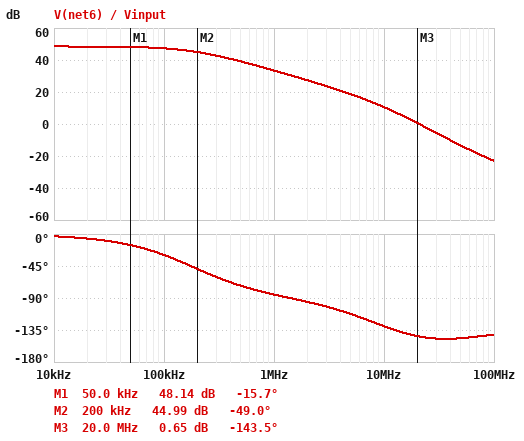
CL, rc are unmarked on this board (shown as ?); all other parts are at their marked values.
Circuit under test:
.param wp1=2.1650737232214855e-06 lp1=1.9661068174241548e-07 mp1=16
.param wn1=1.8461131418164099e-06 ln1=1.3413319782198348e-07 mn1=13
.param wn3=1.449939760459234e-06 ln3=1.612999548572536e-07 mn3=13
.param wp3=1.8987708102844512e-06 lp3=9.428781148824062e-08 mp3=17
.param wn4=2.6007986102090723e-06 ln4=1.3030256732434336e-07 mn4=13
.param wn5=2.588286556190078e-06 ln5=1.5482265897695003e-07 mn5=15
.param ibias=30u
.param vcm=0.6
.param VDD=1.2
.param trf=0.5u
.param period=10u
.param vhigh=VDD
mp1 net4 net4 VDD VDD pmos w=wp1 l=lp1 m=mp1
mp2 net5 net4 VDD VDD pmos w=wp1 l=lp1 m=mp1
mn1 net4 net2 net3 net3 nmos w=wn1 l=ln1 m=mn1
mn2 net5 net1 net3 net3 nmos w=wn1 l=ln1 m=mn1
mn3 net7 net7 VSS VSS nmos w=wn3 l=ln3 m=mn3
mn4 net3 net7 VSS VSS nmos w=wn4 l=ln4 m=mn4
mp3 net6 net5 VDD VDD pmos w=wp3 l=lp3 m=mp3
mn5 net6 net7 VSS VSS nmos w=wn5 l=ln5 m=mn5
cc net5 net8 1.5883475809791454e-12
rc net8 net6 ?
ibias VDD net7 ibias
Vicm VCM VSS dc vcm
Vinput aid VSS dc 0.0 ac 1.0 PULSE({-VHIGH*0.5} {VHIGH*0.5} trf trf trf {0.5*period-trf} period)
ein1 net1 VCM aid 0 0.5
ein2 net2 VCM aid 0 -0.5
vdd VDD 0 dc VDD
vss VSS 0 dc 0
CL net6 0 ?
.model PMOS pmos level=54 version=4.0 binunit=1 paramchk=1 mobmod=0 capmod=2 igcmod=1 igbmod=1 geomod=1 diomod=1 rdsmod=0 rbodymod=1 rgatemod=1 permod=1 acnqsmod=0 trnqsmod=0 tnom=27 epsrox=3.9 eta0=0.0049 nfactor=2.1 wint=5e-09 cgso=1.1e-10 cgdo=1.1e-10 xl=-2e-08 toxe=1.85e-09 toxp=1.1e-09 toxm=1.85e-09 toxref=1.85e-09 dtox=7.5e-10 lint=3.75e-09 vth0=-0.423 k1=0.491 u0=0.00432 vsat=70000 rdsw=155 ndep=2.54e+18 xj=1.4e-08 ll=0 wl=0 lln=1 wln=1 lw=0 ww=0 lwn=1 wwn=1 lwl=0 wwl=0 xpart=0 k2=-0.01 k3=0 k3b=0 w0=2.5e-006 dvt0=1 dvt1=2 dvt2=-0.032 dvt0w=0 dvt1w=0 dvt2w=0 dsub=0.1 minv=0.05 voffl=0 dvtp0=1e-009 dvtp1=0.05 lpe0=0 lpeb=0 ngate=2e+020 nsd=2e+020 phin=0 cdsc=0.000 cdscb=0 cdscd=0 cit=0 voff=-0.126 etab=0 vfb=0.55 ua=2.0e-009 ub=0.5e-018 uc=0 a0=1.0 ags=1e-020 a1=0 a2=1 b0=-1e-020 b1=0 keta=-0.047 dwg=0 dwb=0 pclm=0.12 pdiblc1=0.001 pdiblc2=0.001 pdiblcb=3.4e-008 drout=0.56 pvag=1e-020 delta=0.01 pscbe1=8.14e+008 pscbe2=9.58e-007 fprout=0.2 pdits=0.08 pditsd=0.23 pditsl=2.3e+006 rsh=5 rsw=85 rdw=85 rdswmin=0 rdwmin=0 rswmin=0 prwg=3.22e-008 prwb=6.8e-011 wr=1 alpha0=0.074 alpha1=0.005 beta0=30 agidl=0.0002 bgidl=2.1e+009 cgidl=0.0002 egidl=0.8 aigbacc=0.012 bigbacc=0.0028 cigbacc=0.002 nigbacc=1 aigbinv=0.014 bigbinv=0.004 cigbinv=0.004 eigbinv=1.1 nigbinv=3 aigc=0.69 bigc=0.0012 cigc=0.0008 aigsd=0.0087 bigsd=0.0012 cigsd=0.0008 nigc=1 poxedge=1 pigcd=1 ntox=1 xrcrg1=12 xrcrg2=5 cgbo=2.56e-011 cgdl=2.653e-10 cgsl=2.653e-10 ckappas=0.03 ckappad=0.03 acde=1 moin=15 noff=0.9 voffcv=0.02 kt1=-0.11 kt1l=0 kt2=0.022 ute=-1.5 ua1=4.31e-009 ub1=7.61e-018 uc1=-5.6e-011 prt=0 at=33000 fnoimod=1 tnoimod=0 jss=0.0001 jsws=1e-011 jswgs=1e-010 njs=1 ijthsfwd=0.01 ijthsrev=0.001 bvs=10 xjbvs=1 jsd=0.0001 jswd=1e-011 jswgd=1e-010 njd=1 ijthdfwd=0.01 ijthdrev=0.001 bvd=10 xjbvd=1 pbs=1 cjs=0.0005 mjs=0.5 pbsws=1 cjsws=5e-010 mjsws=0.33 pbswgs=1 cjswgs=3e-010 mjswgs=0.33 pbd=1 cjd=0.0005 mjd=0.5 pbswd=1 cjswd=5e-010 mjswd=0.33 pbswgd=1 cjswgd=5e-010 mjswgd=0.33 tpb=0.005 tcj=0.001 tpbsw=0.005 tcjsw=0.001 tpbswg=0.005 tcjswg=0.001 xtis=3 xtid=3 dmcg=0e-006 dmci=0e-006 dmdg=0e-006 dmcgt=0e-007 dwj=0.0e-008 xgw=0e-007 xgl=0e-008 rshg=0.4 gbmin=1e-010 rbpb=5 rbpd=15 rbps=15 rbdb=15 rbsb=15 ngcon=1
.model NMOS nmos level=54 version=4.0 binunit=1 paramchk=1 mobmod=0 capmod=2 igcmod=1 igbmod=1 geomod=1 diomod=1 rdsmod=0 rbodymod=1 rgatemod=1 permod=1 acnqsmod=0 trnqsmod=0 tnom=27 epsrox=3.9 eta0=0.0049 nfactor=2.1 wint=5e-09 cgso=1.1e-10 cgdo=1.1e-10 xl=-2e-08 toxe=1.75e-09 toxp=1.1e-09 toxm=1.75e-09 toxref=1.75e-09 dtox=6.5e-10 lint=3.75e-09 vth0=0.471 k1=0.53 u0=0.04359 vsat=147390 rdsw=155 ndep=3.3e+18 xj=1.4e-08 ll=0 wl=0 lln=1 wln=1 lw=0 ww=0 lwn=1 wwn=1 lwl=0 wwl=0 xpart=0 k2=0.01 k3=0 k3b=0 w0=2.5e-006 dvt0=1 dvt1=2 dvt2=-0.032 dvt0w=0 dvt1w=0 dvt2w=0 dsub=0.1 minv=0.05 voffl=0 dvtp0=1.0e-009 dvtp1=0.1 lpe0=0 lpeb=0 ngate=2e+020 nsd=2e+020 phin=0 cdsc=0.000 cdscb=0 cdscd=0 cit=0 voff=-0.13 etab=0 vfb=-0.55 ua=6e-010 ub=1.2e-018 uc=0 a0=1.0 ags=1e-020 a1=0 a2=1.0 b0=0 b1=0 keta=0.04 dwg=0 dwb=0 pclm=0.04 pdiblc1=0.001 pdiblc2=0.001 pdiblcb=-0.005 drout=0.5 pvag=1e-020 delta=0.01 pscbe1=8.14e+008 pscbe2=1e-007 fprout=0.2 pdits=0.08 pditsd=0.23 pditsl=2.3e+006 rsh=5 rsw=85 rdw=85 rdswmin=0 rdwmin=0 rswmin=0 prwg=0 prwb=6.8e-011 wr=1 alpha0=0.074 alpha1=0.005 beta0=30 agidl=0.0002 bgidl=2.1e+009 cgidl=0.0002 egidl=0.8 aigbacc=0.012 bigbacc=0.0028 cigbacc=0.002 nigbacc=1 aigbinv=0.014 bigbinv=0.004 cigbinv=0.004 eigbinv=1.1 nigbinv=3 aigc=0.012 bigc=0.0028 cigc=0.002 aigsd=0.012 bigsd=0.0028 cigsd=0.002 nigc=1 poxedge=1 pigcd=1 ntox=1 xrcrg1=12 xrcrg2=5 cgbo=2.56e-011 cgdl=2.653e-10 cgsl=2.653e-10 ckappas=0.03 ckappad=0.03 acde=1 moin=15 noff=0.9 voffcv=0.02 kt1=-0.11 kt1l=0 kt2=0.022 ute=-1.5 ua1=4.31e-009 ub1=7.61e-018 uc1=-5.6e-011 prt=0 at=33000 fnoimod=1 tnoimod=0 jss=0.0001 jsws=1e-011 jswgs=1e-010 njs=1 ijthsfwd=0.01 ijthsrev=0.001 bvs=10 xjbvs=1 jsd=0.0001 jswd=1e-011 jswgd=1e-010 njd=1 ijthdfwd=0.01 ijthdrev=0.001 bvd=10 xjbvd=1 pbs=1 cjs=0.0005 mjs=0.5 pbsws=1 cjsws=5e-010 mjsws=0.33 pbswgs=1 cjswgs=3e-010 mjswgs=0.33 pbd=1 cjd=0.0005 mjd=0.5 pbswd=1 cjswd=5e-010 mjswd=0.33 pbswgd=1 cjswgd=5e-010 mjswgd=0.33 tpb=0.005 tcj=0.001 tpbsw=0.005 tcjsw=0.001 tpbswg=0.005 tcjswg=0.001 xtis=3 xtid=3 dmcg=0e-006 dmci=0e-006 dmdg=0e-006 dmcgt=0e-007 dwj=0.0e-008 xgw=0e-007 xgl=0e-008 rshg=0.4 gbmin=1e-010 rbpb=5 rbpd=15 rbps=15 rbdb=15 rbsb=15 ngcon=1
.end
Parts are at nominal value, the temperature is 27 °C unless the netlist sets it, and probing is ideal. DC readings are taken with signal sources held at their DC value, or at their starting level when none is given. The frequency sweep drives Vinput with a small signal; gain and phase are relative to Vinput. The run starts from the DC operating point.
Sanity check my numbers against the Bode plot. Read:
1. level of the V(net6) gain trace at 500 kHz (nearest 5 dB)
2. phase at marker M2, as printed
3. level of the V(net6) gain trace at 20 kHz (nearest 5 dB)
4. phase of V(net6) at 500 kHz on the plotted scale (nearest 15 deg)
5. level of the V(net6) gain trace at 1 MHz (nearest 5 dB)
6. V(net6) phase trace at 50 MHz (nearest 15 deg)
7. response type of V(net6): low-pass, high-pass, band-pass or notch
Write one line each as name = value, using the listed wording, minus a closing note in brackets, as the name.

level of the V(net6) gain trace at 500 kHz = 40 dB
phase at marker M2, as printed = -49.0 deg
level of the V(net6) gain trace at 20 kHz = 50 dB
phase of V(net6) at 500 kHz on the plotted scale = -75 deg
level of the V(net6) gain trace at 1 MHz = 35 dB
V(net6) phase trace at 50 MHz = -150 deg
response type of V(net6): low-pass, high-pass, band-pass or notch = low-pass
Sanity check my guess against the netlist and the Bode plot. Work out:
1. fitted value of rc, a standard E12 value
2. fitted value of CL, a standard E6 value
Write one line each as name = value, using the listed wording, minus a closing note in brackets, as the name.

fitted value of rc, a standard E12 value = 2.2 kΩ
fitted value of CL, a standard E6 value = 22 pF
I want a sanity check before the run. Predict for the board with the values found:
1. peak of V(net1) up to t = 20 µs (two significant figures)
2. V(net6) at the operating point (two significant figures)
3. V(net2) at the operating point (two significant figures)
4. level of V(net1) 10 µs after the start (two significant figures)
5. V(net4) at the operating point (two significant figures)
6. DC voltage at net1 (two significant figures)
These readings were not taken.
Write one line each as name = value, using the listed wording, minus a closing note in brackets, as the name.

peak of V(net1) up to t = 20 µs = 900 mV
V(net6) at the operating point = 1.1 V
V(net2) at the operating point = 600 mV
level of V(net1) 10 µs after the start = 300 mV
V(net4) at the operating point = 720 mV
DC voltage at net1 = 600 mV
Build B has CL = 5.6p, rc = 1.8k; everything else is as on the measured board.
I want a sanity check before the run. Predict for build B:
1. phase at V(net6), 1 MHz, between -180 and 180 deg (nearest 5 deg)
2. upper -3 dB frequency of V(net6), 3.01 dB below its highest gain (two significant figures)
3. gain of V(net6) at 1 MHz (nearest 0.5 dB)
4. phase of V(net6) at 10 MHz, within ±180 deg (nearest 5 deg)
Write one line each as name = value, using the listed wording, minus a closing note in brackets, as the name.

phase at V(net6), 1 MHz, between -180 and 180 deg = -80 deg
upper -3 dB frequency of V(net6), 3.01 dB below its highest gain = 190 kHz
gain of V(net6) at 1 MHz = 34.0 dB
phase of V(net6) at 10 MHz, within ±180 deg = -100 deg
